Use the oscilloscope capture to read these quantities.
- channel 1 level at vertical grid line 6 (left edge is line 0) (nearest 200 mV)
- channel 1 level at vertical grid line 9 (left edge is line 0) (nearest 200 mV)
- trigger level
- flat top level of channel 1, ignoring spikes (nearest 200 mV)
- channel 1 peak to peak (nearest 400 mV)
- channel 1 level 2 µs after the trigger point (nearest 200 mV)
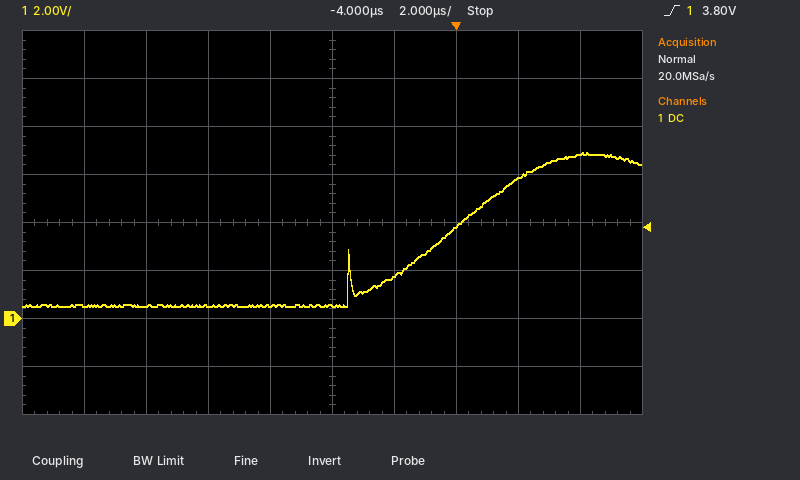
1.8 V
6.8 V
3.80 V
6.8 V
6.4 V
5.8 V
